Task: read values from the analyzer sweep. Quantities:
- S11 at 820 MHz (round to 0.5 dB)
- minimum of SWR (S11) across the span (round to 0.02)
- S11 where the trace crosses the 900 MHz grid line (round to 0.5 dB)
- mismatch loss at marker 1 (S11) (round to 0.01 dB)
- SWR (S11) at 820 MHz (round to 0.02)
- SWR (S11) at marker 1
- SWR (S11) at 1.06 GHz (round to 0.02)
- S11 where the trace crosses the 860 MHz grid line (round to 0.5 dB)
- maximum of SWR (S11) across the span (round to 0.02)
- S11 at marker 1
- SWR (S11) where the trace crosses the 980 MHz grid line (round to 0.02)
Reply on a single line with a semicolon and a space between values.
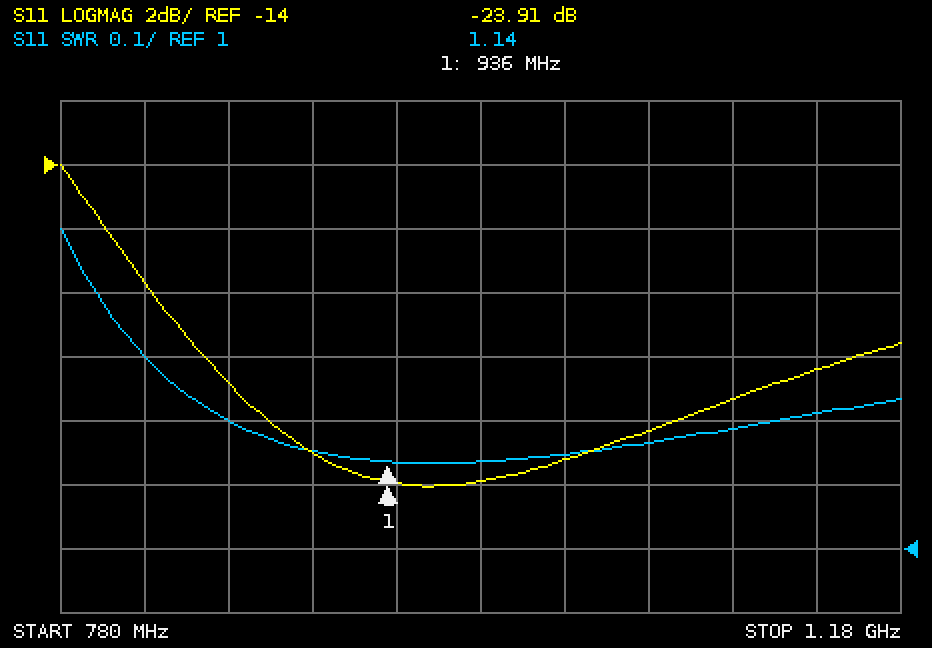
-17.5 dB; 1.14; -23.0 dB; 0.02 dB; 1.30; 1.14; 1.16; -21.0 dB; 1.50; -23.91 dB; 1.14
